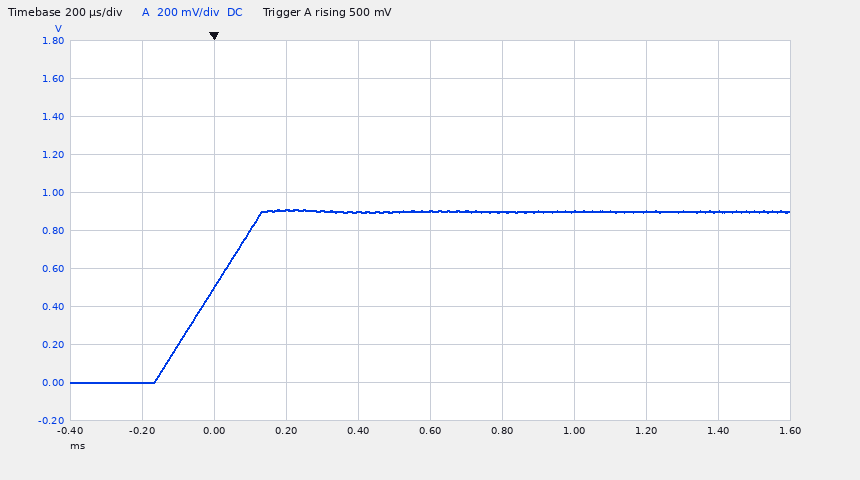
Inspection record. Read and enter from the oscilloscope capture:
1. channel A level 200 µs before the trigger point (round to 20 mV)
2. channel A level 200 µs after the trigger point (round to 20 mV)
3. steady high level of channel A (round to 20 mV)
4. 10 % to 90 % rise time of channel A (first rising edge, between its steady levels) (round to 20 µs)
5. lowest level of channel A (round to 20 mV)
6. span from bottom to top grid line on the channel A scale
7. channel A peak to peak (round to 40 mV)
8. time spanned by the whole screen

0 mV
900 mV
900 mV
240 µs
0 mV
2 V
920 mV
2 ms
